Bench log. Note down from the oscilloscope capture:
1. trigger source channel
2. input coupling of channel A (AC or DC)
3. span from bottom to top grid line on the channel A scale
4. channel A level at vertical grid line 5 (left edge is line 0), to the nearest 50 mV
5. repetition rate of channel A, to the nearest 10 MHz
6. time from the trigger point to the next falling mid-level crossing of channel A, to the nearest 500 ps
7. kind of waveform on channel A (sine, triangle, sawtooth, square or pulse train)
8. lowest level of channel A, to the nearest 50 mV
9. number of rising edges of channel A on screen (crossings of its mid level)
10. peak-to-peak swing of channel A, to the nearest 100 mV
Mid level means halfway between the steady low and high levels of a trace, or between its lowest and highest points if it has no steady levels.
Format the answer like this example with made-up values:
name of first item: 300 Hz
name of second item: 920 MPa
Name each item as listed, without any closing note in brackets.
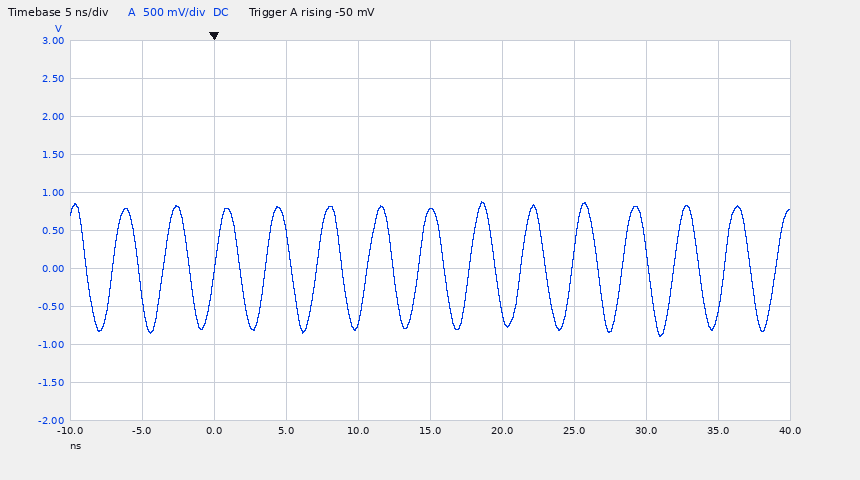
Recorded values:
trigger source channel: channel A
input coupling of channel A: DC
span from bottom to top grid line on the channel A scale: 5 V
channel A level at vertical grid line 5 (left edge is line 0), to the nearest 50 mV: 750 mV
repetition rate of channel A, to the nearest 10 MHz: 280 MHz
time from the trigger point to the next falling mid-level crossing of channel A, to the nearest 500 ps: 2.0 ns
kind of waveform on channel A: sine
lowest level of channel A, to the nearest 50 mV: -900 mV
number of rising edges of channel A on screen: 14
peak-to-peak swing of channel A, to the nearest 100 mV: 1.80 V
